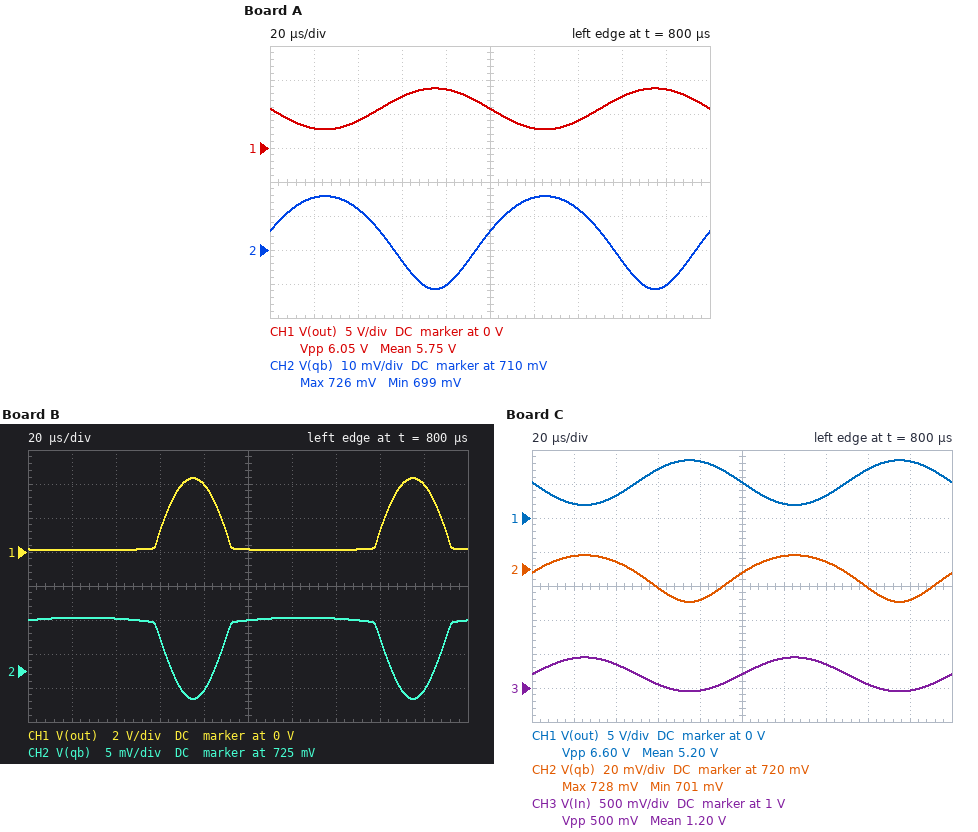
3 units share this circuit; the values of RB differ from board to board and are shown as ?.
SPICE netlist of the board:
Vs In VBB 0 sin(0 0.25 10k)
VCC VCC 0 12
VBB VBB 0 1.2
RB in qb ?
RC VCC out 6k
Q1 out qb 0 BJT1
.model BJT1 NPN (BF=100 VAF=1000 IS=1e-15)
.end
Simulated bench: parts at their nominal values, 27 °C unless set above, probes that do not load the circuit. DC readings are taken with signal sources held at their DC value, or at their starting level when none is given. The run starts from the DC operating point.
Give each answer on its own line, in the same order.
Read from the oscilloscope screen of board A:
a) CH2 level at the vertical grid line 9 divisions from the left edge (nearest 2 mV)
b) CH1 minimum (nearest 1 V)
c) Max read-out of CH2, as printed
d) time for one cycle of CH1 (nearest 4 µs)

700 mV
3 V
726 mV
100 µs
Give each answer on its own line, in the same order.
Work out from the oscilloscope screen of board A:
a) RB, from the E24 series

47 kΩ
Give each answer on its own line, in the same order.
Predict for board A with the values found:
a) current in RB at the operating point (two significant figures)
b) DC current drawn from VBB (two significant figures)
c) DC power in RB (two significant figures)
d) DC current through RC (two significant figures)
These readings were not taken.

10 µA
10 µA
5.0 µW
1.0 mA
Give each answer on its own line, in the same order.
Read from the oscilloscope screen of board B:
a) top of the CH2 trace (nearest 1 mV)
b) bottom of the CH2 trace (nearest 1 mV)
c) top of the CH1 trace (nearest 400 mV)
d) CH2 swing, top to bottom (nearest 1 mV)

733 mV
721 mV
4.4 V
12 mV
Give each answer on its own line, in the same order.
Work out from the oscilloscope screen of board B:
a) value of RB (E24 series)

18 kΩ
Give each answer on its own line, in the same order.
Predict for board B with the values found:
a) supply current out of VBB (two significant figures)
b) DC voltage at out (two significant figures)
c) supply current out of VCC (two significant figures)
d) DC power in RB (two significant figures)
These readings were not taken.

26 µA
150 mV
2.0 mA
12 µW
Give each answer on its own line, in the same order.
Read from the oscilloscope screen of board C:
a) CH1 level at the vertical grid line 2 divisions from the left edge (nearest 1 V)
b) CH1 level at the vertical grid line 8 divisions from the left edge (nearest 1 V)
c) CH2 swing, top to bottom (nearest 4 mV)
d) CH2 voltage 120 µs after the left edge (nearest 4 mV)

3 V
7 V
28 mV
728 mV
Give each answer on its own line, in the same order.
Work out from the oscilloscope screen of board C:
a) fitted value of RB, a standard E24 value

43 kΩ
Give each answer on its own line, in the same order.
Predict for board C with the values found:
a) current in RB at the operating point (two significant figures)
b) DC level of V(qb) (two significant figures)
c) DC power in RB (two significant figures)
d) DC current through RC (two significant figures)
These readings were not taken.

11 µA
720 mV
5.4 µW
1.1 mA
